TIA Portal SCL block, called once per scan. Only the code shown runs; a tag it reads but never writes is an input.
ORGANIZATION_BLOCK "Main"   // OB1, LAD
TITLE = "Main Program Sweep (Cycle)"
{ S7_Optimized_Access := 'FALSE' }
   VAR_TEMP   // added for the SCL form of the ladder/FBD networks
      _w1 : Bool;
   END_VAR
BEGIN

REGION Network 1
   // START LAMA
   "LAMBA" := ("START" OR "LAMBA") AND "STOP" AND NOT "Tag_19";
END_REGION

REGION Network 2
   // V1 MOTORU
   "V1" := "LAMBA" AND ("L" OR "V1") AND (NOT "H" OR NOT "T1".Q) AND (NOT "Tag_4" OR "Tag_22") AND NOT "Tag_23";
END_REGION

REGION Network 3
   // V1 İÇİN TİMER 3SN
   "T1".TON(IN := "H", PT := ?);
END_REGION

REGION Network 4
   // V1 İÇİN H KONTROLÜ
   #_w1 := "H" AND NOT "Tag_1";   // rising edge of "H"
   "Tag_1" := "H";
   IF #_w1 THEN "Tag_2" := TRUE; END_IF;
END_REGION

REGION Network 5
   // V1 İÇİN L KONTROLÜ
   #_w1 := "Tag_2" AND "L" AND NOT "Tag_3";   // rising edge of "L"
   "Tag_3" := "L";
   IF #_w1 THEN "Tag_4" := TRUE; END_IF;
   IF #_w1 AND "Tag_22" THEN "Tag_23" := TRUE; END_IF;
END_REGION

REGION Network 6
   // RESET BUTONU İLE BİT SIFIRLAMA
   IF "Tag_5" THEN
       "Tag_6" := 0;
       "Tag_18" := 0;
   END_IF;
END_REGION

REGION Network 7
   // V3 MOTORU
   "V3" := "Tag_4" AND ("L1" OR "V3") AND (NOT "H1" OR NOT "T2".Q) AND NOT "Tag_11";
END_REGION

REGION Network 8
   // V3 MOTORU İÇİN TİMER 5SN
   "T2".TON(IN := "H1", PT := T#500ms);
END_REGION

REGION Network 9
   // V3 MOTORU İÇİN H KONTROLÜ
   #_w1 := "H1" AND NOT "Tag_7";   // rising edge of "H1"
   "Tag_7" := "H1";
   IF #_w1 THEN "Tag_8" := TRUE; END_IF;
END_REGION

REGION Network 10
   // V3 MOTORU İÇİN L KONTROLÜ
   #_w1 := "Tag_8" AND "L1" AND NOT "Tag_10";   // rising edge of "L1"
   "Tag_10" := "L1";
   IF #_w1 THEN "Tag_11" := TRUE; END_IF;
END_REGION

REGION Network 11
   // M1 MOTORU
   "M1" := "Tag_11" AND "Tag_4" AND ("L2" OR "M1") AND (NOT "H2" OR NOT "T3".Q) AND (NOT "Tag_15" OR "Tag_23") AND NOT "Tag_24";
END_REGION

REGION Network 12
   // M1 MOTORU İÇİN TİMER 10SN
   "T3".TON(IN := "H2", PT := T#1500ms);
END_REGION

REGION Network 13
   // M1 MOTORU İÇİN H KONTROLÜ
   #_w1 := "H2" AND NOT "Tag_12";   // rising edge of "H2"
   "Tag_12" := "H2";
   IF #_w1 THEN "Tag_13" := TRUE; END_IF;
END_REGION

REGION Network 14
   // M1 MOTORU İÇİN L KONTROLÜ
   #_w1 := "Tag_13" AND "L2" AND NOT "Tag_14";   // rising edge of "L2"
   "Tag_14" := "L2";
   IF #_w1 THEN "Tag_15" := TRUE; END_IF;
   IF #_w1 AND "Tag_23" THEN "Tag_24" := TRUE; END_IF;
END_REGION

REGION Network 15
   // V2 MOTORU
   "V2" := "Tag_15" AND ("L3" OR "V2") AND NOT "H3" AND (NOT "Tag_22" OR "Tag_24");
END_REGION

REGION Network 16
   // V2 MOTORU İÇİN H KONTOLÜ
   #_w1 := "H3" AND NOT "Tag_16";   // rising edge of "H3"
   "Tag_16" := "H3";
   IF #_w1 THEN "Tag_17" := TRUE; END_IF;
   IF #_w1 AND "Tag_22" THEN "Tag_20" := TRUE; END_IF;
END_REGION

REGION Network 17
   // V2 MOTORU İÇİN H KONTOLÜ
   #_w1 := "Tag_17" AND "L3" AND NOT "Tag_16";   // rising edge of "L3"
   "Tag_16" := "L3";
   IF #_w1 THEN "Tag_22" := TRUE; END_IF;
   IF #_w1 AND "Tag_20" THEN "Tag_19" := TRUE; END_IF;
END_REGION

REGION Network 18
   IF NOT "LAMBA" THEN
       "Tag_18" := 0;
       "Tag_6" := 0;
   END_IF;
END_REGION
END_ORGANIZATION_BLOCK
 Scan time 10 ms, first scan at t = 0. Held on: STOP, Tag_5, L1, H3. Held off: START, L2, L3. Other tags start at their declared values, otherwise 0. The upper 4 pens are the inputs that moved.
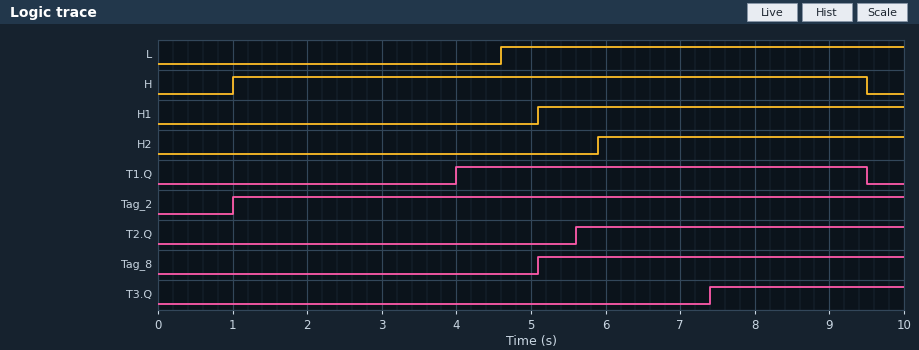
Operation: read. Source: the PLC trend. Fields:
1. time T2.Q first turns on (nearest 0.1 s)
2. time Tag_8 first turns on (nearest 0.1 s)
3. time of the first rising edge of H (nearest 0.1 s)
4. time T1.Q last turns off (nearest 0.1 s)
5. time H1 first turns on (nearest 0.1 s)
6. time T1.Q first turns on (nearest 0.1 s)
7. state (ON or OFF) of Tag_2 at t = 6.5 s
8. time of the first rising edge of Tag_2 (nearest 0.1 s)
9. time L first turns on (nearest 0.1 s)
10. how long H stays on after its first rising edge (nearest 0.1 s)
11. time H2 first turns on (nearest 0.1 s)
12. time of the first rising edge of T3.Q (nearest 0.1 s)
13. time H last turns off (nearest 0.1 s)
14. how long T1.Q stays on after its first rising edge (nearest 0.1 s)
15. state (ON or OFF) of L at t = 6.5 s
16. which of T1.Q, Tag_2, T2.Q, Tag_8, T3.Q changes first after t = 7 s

5.6 s
5.1 s
1.0 s
9.5 s
5.1 s
4.0 s
ON
1.0 s
4.6 s
8.5 s
5.9 s
7.4 s
9.5 s
5.5 s
ON
T3.Q
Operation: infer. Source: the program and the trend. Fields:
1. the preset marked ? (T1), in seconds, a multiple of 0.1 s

3.0 s
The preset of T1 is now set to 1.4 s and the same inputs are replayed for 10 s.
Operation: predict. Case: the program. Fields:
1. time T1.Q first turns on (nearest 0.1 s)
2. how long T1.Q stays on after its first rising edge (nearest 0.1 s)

2.4 s
7.1 s
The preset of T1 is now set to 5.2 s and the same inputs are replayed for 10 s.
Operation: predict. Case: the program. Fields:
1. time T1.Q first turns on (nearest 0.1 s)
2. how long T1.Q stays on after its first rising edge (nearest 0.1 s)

6.2 s
3.3 s
